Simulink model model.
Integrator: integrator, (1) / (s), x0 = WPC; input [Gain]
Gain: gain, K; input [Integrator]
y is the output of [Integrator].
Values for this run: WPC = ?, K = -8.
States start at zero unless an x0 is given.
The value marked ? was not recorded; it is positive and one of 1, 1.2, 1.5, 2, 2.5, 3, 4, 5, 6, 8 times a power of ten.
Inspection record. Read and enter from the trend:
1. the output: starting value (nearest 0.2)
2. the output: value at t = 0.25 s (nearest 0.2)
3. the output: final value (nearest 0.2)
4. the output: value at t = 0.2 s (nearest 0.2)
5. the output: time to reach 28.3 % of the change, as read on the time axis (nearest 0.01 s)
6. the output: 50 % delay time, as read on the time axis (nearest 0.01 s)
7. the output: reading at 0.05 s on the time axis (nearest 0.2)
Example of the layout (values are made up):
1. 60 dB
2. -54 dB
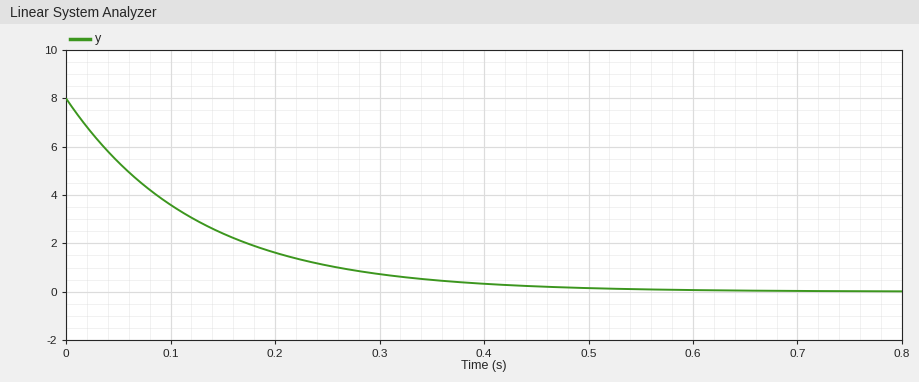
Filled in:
1. 8.0
2. 1.0
3. 0.0
4. 1.6
5. 0.04 s
6. 0.09 s
7. 5.4
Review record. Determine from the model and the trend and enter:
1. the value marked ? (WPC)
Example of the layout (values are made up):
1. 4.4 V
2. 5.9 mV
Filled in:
1. 8
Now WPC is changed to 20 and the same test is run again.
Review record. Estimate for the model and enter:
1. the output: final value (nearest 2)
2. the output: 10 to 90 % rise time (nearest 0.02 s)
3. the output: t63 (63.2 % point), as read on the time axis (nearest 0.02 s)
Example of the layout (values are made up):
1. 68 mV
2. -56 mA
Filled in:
1. 0
2. 0.28 s
3. 0.12 s
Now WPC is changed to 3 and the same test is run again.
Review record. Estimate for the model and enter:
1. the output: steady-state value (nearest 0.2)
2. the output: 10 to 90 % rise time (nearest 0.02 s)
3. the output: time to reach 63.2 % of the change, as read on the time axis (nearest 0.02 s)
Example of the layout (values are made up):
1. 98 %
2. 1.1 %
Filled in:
1. 0.0
2. 0.28 s
3. 0.12 s
